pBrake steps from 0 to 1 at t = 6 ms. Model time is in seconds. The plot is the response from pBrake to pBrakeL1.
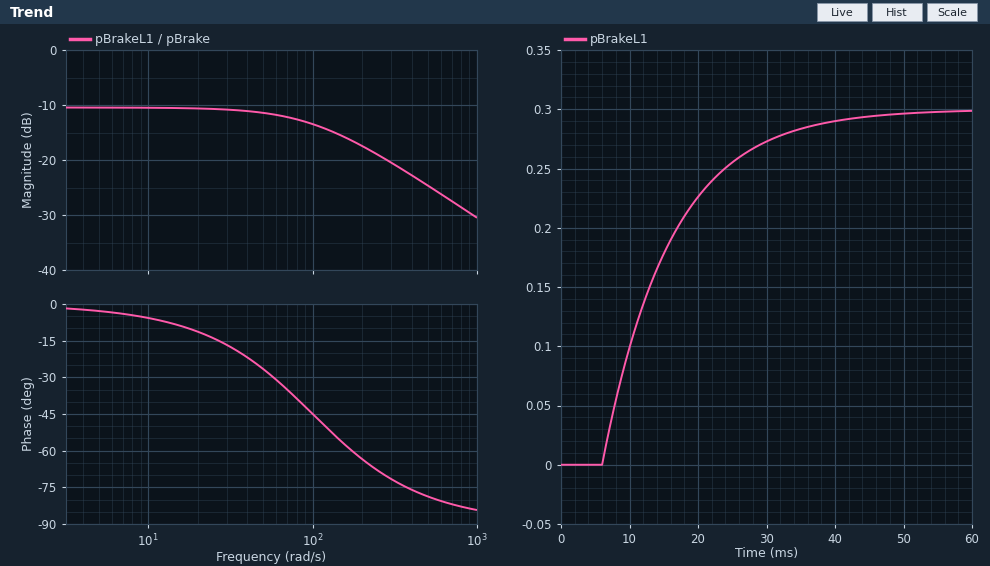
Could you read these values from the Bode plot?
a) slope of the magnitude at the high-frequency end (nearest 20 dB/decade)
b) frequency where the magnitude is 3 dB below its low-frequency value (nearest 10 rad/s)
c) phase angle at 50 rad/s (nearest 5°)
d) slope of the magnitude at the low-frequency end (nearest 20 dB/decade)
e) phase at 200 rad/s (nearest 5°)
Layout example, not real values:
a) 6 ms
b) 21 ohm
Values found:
a) -20 dB/decade
b) 100 rad/s
c) -25°
d) 0 dB/decade
e) -65°
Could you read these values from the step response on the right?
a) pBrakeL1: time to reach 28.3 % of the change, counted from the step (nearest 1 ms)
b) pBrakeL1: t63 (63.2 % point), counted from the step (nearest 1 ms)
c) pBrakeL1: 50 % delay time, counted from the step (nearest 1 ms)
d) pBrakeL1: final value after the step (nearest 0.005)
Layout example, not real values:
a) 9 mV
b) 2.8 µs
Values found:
a) 3 ms
b) 10 ms
c) 7 ms
d) 0.300
